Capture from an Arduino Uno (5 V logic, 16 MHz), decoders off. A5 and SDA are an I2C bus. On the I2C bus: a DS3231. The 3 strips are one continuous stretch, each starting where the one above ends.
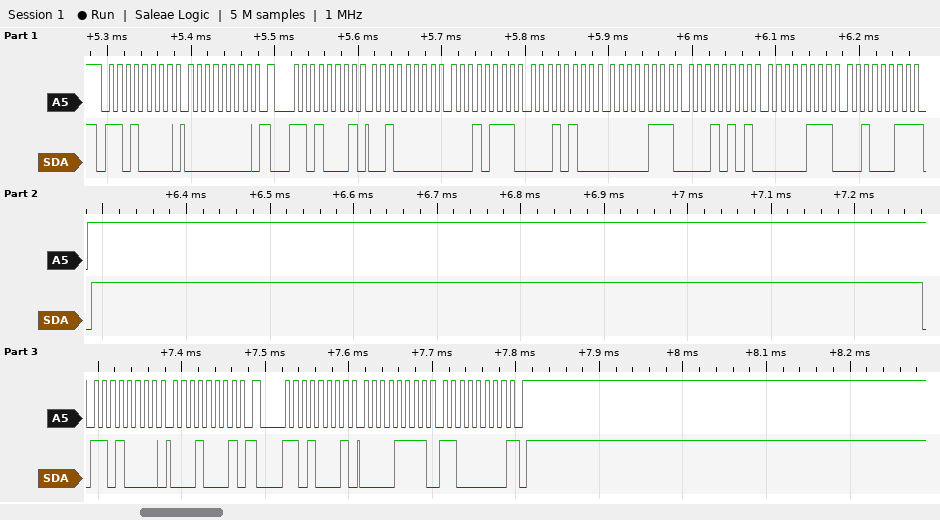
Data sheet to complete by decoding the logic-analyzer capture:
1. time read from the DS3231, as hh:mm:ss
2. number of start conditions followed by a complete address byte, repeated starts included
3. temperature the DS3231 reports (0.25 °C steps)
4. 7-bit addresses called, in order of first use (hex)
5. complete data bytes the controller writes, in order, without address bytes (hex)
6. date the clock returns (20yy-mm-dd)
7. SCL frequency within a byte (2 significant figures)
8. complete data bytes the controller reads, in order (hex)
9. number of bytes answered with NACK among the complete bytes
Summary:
14:17:20
4
15.75 °C
0x68
00 11
2023-07-15
100 kHz
20 17 14 07 15 07 23 0F C0
2
